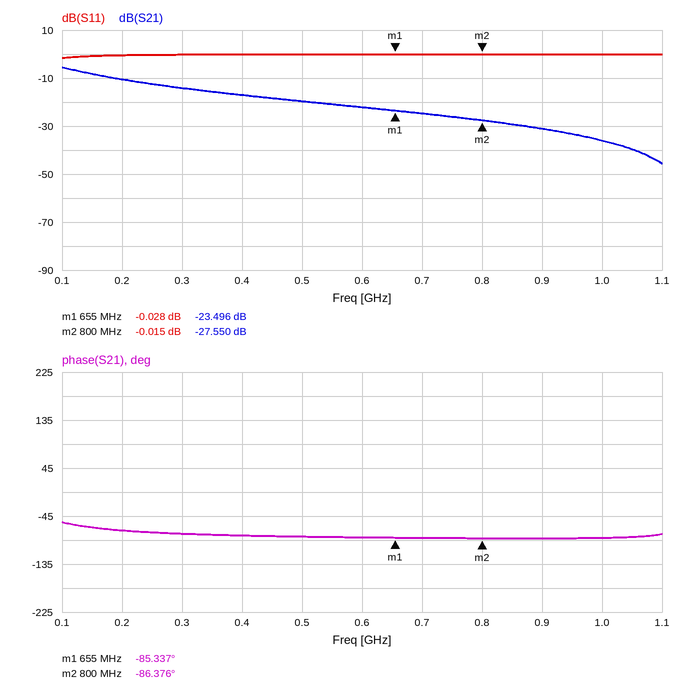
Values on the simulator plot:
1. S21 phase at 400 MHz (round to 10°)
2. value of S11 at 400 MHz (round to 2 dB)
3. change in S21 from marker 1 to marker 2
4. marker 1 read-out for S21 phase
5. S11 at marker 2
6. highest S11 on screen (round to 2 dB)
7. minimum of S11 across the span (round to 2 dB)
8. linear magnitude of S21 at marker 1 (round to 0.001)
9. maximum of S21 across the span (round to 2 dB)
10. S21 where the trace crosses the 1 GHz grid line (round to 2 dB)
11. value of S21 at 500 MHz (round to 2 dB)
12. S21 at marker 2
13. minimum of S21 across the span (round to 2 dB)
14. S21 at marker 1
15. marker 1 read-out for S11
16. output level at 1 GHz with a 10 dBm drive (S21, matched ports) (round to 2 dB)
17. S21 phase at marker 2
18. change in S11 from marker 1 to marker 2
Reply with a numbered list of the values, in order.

1. -80°
2. 0 dB
3. -4.054 dB
4. -85.337°
5. -0.015 dB
6. 0 dB
7. -2 dB
8. 0.067
9. -6 dB
10. -36 dB
11. -20 dB
12. -27.550 dB
13. -46 dB
14. -23.496 dB
15. -0.028 dB
16. -26 dBm
17. -86.376°
18. 0.013 dB
